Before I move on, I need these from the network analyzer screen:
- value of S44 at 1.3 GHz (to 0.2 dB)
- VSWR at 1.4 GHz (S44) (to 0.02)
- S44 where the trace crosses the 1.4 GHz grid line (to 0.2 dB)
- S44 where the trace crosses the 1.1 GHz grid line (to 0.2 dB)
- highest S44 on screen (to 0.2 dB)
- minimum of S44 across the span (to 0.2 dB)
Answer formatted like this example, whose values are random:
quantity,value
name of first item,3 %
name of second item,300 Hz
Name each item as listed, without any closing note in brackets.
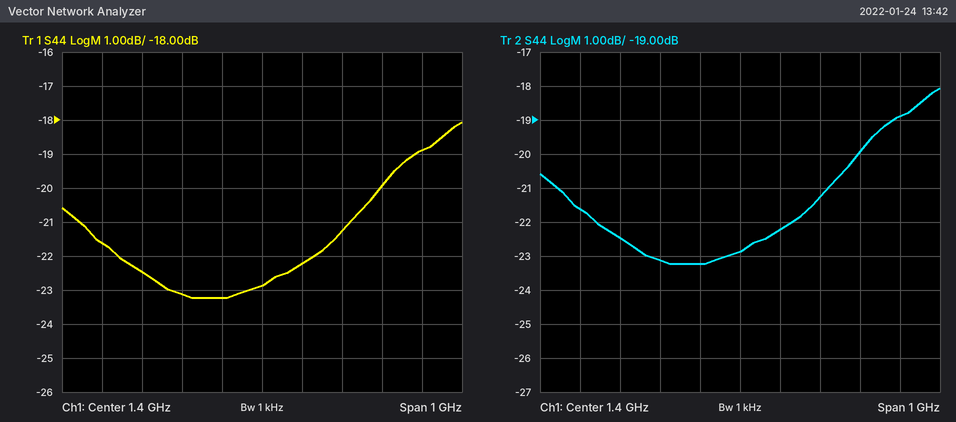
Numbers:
quantity,value
value of S44 at 1.3 GHz,-23.2 dB
VSWR at 1.4 GHz (S44),1.16
S44 where the trace crosses the 1.4 GHz grid line,-22.8 dB
S44 where the trace crosses the 1.1 GHz grid line,-22.4 dB
highest S44 on screen,-18.0 dB
minimum of S44 across the span,-23.2 dB
